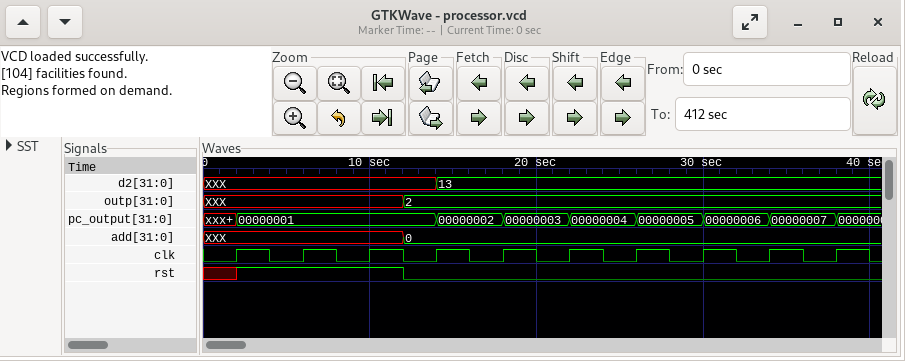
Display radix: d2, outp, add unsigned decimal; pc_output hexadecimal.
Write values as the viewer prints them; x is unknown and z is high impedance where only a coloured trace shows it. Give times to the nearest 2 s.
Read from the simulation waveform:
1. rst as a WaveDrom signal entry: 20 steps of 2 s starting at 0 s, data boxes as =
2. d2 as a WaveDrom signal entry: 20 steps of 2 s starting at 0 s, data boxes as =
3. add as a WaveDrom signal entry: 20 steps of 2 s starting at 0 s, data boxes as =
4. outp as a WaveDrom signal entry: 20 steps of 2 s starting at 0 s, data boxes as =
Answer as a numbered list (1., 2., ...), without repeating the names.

1. {name: 'rst', wave: 'x1....0.............'}
2. {name: 'd2', wave: 'x......=............', data: '13'}
3. {name: 'add', wave: 'x.....=.............', data: '0'}
4. {name: 'outp', wave: '=.....=.............', data: 'XXX 2'}
